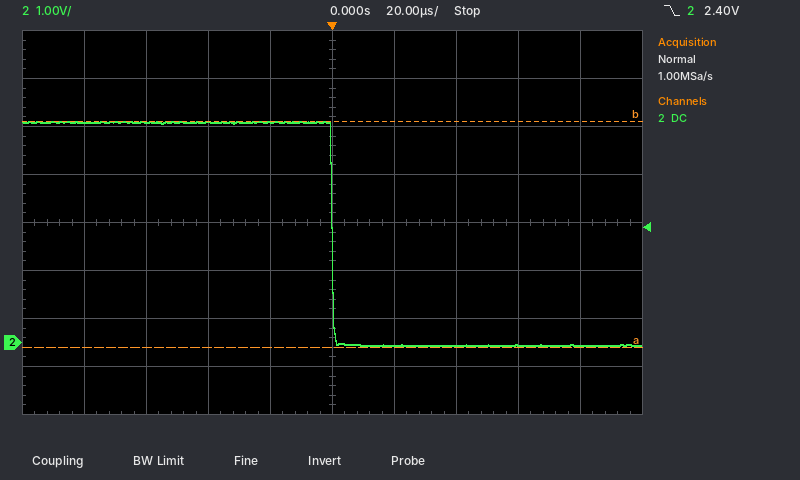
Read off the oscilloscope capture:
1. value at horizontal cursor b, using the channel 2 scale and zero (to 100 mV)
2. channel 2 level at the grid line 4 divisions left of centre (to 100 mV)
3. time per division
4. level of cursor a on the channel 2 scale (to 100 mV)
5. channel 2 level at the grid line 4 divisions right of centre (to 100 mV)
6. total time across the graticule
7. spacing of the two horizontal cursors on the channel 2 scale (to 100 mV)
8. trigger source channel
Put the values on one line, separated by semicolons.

4.6 V; 4.6 V; 20 µs; -100 mV; -100 mV; 200 µs; 4.7 V; channel 2
